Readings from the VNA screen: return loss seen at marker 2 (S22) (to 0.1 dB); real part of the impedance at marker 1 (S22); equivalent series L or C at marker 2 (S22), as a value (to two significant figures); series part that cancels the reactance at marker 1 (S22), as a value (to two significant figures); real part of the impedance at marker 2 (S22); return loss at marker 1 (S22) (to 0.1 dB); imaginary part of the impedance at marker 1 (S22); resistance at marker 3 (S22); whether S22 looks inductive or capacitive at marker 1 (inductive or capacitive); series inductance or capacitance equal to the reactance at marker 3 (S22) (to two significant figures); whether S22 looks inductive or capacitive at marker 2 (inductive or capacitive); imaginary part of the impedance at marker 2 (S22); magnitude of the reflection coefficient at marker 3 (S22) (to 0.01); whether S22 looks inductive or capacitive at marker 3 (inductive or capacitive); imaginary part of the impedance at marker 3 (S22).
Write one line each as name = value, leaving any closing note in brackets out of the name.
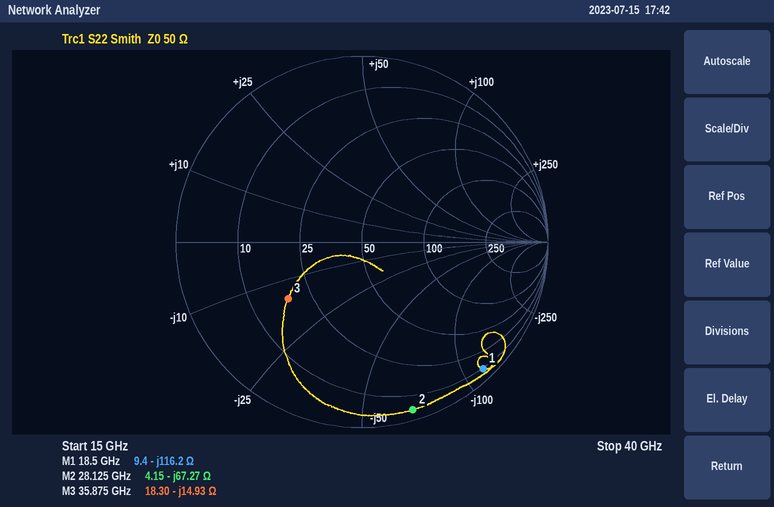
return loss seen at marker 2 (S22) = 0.5 dB
real part of the impedance at marker 1 = 9.4 Ω
equivalent series L or C at marker 2 (S22), as a value = 84 fF
series part that cancels the reactance at marker 1 (S22), as a value = 1.00 nH
real part of the impedance at marker 2 = 4.15 Ω
return loss at marker 1 (S22) = 0.5 dB
imaginary part of the impedance at marker 1 = -116.2 Ω
resistance at marker 3 = 18.30 Ω
whether S22 looks inductive or capacitive at marker 1 = capacitive
series inductance or capacitance equal to the reactance at marker 3 (S22) = 300 fF
whether S22 looks inductive or capacitive at marker 2 = capacitive
imaginary part of the impedance at marker 2 = -67.27 Ω
magnitude of the reflection coefficient at marker 3 (S22) = 0.50
whether S22 looks inductive or capacitive at marker 3 = capacitive
imaginary part of the impedance at marker 3 = -14.93 Ω
